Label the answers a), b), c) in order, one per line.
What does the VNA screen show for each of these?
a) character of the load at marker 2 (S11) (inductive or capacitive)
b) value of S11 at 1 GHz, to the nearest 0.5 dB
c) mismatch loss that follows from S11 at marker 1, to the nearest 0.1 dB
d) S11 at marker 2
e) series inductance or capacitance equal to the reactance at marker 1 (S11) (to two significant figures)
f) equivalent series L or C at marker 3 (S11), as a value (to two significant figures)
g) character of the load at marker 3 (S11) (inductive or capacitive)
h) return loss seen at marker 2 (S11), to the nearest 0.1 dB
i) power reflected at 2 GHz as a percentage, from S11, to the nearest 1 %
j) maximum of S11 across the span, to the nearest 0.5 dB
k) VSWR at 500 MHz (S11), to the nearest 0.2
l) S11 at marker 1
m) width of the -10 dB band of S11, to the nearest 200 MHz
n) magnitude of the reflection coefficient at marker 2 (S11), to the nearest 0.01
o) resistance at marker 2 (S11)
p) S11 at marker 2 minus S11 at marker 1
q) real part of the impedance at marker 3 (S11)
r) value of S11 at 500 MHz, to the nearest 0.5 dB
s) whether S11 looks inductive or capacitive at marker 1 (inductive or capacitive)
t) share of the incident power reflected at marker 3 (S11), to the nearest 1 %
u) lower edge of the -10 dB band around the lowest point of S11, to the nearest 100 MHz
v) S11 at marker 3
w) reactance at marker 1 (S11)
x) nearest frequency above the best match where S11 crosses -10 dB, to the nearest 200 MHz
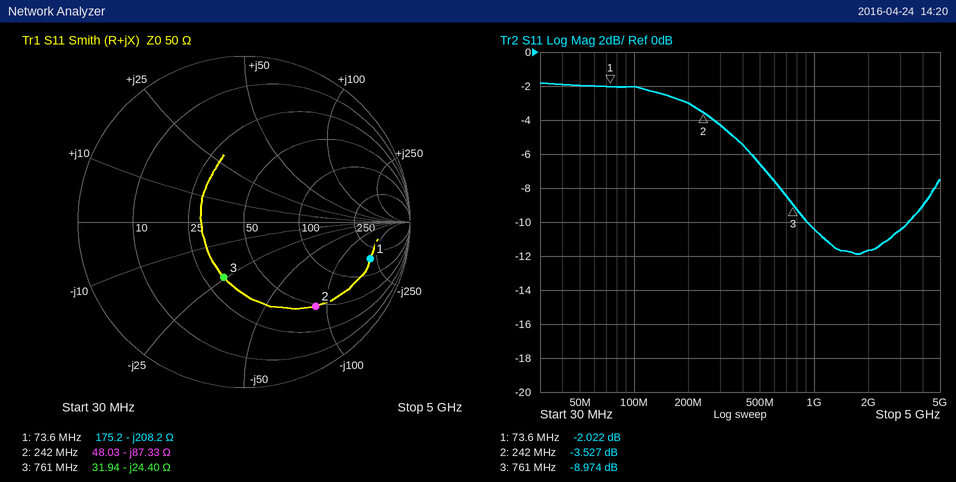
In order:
a) capacitive
b) -10.5 dB
c) 4.3 dB
d) -3.527 dB
e) 10 pF
f) 8.6 pF
g) capacitive
h) 3.5 dB
i) 7 %
j) -2.0 dB
k) 2.8
l) -2.022 dB
m) 2.4 GHz
n) 0.67
o) 48.03 Ω
p) -1.505 dB
q) 31.94 Ω
r) -6.5 dB
s) capacitive
t) 13 %
u) 900 MHz
v) -8.974 dB
w) -208.2 Ω
x) 3.4 GHz
